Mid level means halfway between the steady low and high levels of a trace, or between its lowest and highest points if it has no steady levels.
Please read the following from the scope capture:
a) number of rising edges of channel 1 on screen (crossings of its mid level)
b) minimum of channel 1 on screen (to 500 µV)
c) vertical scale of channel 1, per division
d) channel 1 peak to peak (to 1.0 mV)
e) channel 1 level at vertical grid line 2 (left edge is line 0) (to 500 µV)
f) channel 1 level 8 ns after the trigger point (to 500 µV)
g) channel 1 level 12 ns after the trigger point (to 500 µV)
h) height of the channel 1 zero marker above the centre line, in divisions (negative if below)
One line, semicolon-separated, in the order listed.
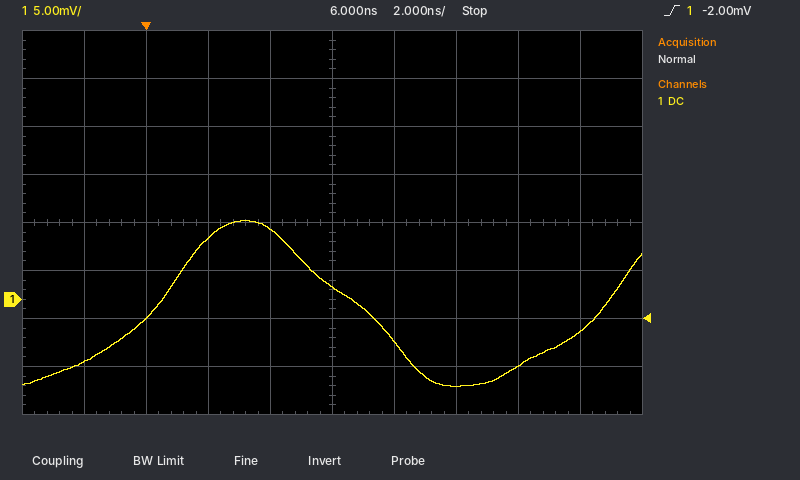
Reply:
2; -9.0 mV; 5 mV; 17.0 mV; -2.0 mV; -4.5 mV; -7.0 mV; -1.6 div
